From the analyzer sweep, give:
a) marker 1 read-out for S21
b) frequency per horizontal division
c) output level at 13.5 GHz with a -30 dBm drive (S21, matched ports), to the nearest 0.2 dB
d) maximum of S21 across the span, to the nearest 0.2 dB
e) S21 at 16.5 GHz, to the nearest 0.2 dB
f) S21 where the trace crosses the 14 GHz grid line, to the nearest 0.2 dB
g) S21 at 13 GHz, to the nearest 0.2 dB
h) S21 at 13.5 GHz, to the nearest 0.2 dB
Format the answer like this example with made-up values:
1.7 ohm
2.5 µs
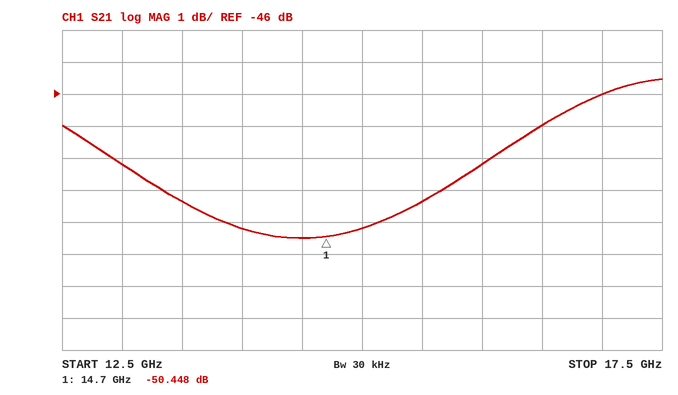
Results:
-50.448 dB
500 MHz
-79.4 dBm
-45.6 dB
-47.0 dB
-50.2 dB
-48.2 dB
-49.4 dB
